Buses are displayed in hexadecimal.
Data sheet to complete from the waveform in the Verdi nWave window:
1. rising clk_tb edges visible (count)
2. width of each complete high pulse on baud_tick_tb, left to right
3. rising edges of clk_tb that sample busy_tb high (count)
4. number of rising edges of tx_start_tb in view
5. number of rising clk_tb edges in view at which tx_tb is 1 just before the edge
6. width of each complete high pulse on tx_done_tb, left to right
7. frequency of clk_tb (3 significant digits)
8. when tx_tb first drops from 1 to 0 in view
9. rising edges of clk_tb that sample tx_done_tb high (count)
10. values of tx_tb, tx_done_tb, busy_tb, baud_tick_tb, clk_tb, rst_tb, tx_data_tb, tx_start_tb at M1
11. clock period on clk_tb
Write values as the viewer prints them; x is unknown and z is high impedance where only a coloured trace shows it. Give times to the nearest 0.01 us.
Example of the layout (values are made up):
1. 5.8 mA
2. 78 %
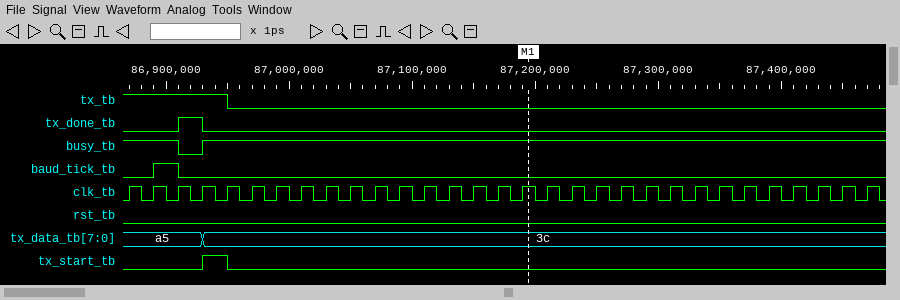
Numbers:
1. 31
2. 0.02 us
3. 30
4. 1
5. 5
6. 0.02 us
7. 50.0 MHz
8. 86.95 us
9. 1
10. tx_tb=0, tx_done_tb=0, busy_tb=1, baud_tick_tb=0, clk_tb=1, rst_tb=0, tx_data_tb=3c, tx_start_tb=0
11. 0.02 us
